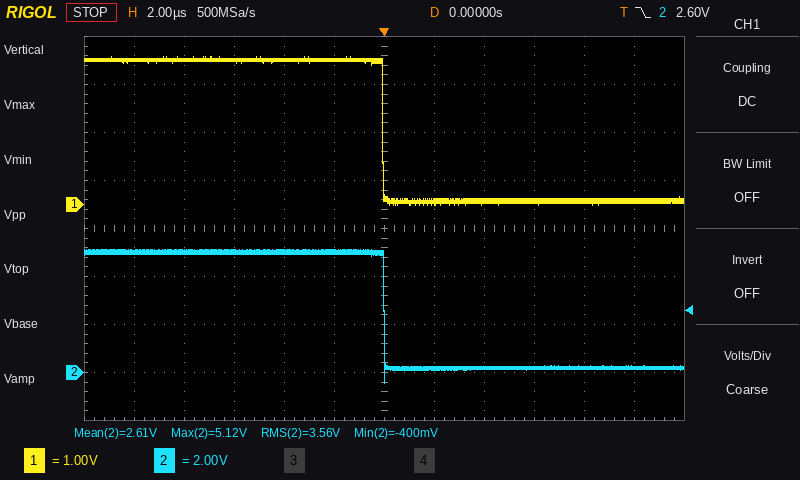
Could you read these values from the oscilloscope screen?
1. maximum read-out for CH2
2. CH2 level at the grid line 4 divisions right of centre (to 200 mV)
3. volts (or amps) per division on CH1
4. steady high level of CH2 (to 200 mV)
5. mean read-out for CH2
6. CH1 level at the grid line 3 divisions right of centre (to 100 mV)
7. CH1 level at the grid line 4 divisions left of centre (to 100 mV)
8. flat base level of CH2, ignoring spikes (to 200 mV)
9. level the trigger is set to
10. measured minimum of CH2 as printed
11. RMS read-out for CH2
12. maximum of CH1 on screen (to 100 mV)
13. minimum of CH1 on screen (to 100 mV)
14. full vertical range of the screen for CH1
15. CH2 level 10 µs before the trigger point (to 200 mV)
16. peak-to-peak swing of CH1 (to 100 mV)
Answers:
5.12 V
200 mV
1 V
5.0 V
2.61 V
100 mV
3.0 V
200 mV
2.60 V
-400 mV
3.56 V
3.1 V
0.0 V
8 V
5.0 V
3.1 V
